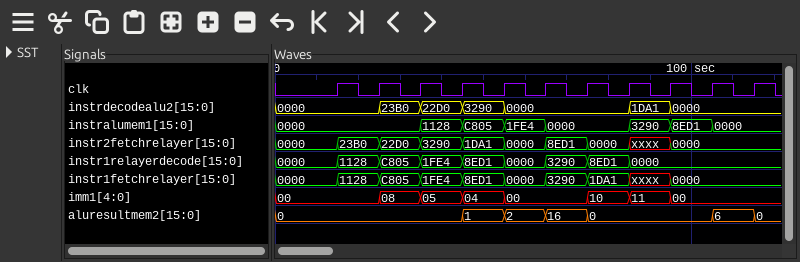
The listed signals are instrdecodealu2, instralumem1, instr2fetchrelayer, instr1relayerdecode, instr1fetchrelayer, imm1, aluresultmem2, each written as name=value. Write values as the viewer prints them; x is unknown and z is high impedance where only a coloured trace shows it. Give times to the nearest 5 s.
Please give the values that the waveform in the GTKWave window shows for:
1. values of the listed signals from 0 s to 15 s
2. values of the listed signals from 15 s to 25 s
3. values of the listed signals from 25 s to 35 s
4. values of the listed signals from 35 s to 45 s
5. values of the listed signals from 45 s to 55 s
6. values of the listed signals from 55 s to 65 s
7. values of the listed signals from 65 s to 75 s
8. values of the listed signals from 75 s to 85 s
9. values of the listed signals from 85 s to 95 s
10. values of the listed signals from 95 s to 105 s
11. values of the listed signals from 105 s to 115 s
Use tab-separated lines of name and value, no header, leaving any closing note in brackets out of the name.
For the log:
values of the listed signals from 0 s to 15 s	instrdecodealu2=0000, instralumem1=0000, instr2fetchrelayer=0000, instr1relayerdecode=0000, instr1fetchrelayer=0000, imm1=00, aluresultmem2=0
values of the listed signals from 15 s to 25 s	instrdecodealu2=0000, instralumem1=0000, instr2fetchrelayer=23B0, instr1relayerdecode=1128, instr1fetchrelayer=1128, imm1=00, aluresultmem2=0
values of the listed signals from 25 s to 35 s	instrdecodealu2=23B0, instralumem1=0000, instr2fetchrelayer=22D0, instr1relayerdecode=C805, instr1fetchrelayer=C805, imm1=08, aluresultmem2=0
values of the listed signals from 35 s to 45 s	instrdecodealu2=22D0, instralumem1=1128, instr2fetchrelayer=3290, instr1relayerdecode=1FE4, instr1fetchrelayer=1FE4, imm1=05, aluresultmem2=0
values of the listed signals from 45 s to 55 s	instrdecodealu2=3290, instralumem1=C805, instr2fetchrelayer=1DA1, instr1relayerdecode=8ED1, instr1fetchrelayer=8ED1, imm1=04, aluresultmem2=1
values of the listed signals from 55 s to 65 s	instrdecodealu2=0000, instralumem1=1FE4, instr2fetchrelayer=0000, instr1relayerdecode=0000, instr1fetchrelayer=0000, imm1=00, aluresultmem2=2
values of the listed signals from 65 s to 75 s	instrdecodealu2=0000, instralumem1=0000, instr2fetchrelayer=8ED1, instr1relayerdecode=3290, instr1fetchrelayer=3290, imm1=00, aluresultmem2=16
values of the listed signals from 75 s to 85 s	instrdecodealu2=0000, instralumem1=0000, instr2fetchrelayer=0000, instr1relayerdecode=8ED1, instr1fetchrelayer=1DA1, imm1=10, aluresultmem2=0
values of the listed signals from 85 s to 95 s	instrdecodealu2=1DA1, instralumem1=3290, instr2fetchrelayer=xxxx, instr1relayerdecode=0000, instr1fetchrelayer=xxxx, imm1=11, aluresultmem2=0
values of the listed signals from 95 s to 105 s	instrdecodealu2=0000, instralumem1=8ED1, instr2fetchrelayer=0000, instr1relayerdecode=0000, instr1fetchrelayer=0000, imm1=00, aluresultmem2=0
values of the listed signals from 105 s to 115 s	instrdecodealu2=0000, instralumem1=0000, instr2fetchrelayer=0000, instr1relayerdecode=0000, instr1fetchrelayer=0000, imm1=00, aluresultmem2=6
